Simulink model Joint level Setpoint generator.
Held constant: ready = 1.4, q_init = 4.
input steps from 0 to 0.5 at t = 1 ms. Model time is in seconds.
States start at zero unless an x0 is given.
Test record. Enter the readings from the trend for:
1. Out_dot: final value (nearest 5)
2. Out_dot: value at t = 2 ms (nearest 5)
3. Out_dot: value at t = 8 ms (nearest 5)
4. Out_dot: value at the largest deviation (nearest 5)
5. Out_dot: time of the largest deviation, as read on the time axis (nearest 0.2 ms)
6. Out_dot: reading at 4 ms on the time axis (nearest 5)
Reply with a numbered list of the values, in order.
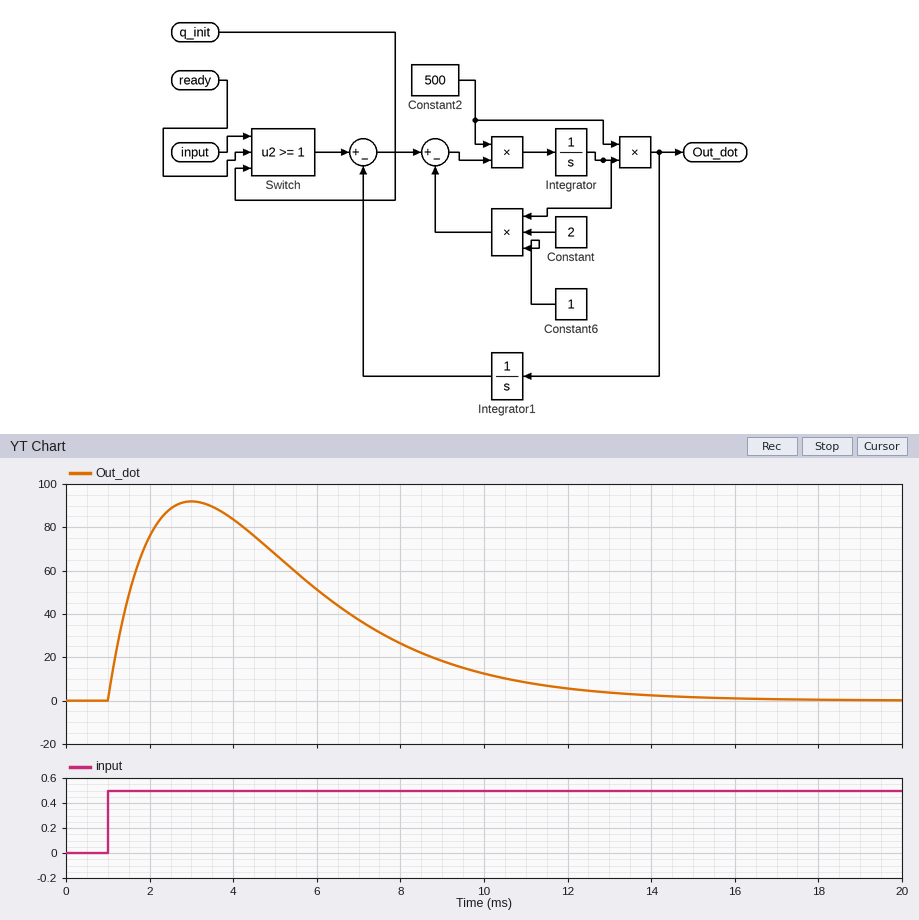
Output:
1. 0
2. 75
3. 25
4. 90
5. 3.0 ms
6. 85
